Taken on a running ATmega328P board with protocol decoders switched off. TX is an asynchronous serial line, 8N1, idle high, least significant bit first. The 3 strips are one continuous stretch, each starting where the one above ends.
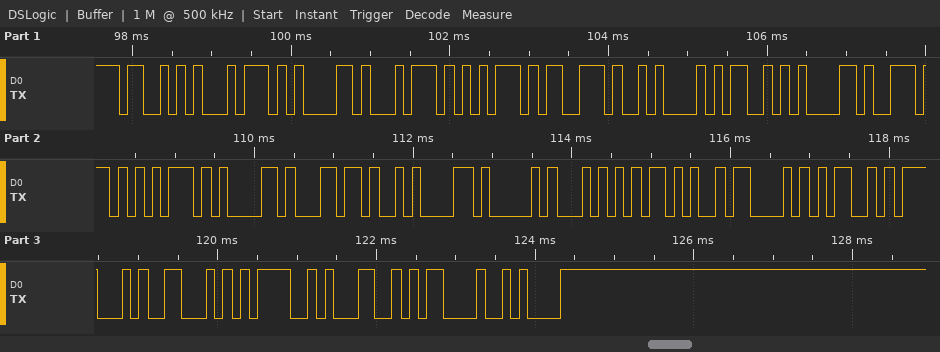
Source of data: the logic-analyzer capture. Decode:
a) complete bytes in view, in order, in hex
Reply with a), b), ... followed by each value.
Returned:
a) 53 74 61 74 75 73 0A 4D 61 6E 75 61 6C 0A 41 54 2B 43 4D 47 46 3D 31 0D 0A
